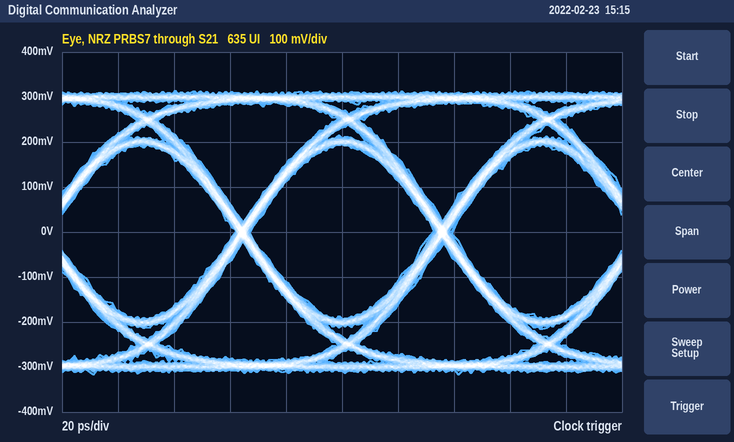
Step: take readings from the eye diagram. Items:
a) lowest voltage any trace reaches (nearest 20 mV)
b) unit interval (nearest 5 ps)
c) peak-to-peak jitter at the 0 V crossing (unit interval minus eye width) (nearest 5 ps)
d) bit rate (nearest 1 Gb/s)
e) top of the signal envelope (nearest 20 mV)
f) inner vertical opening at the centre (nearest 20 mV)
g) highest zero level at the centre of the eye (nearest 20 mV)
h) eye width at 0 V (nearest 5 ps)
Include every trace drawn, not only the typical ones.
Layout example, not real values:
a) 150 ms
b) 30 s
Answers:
a) -320 mV
b) 70 ps
c) 5 ps
d) 14 Gb/s
e) 320 mV
f) 380 mV
g) -200 mV
h) 65 ps
